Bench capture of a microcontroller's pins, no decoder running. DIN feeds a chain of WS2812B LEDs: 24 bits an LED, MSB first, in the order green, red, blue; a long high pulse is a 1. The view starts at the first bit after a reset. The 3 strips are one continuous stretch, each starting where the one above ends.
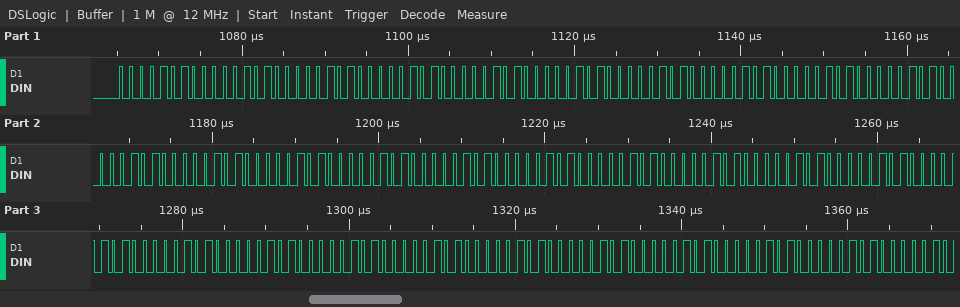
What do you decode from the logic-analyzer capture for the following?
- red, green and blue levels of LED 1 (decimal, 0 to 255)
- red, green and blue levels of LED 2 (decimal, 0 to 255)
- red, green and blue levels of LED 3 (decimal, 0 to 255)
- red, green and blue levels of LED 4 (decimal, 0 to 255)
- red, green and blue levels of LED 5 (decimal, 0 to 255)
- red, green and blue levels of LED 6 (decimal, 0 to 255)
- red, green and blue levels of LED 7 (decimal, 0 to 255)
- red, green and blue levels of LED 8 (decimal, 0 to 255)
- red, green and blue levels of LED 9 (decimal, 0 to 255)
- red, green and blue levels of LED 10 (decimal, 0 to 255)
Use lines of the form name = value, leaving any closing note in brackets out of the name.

red, green and blue levels of LED 1 = 10, 10, 10
red, green and blue levels of LED 2 = 10, 10, 10
red, green and blue levels of LED 3 = 10, 10, 10
red, green and blue levels of LED 4 = 10, 10, 10
red, green and blue levels of LED 5 = 10, 10, 10
red, green and blue levels of LED 6 = 10, 10, 10
red, green and blue levels of LED 7 = 10, 10, 10
red, green and blue levels of LED 8 = 10, 10, 10
red, green and blue levels of LED 9 = 10, 10, 10
red, green and blue levels of LED 10 = 10, 10, 10
